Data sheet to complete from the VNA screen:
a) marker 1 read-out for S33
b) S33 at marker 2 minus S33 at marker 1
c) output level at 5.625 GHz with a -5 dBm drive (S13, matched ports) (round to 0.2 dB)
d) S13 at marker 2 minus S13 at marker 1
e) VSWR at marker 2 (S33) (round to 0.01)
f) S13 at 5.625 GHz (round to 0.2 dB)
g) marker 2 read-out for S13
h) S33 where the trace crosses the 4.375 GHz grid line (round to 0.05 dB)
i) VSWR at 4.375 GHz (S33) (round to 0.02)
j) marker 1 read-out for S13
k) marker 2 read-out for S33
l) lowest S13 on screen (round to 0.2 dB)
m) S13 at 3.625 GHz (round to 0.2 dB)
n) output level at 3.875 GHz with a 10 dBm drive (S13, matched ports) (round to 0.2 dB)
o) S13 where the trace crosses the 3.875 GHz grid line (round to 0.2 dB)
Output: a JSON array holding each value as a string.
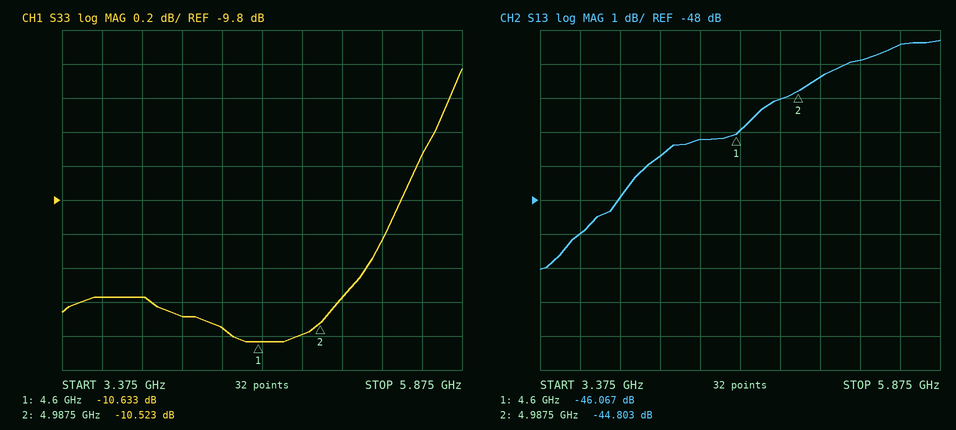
["-10.633 dB", "0.110 dB", "-48.4 dBm", "1.264 dB", "1.85", "-43.4 dB", "-44.803 dB", "-10.55 dB", "1.84", "-46.067 dB", "-10.523 dB", "-50.0 dB", "-49.0 dB", "-38.0 dBm", "-48.0 dB"]
